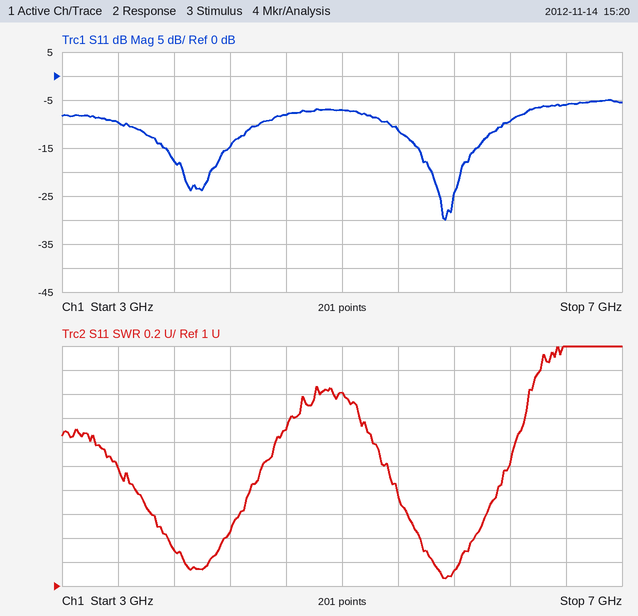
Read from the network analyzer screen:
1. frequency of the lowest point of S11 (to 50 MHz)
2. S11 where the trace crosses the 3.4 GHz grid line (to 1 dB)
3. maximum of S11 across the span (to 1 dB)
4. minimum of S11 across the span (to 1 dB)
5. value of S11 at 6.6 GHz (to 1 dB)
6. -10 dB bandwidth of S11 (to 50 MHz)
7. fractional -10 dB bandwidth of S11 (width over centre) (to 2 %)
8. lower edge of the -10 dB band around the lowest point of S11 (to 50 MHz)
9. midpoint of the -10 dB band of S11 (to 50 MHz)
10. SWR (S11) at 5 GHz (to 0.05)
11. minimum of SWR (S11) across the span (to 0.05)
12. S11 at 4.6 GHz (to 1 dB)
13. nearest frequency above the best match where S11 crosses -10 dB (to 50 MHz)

5.75 GHz
-10 dB
-5 dB
-30 dB
-6 dB
800 MHz
14 %
5.35 GHz
5.75 GHz
2.60
1.05
-8 dB
6.15 GHz
